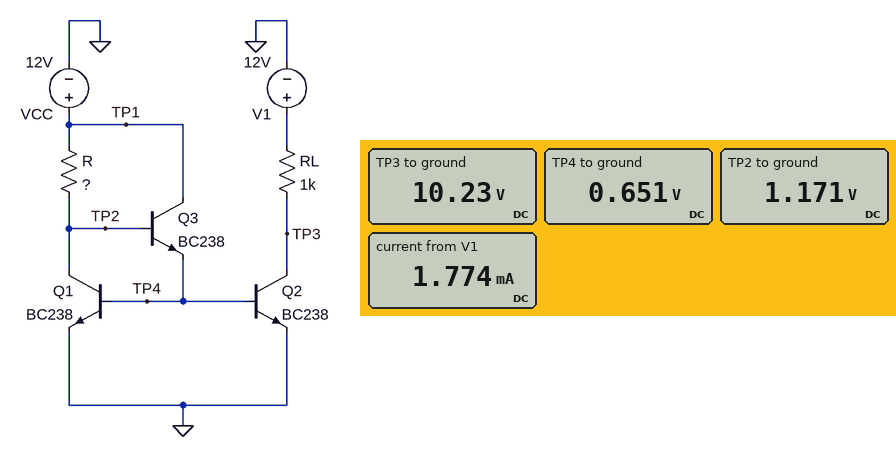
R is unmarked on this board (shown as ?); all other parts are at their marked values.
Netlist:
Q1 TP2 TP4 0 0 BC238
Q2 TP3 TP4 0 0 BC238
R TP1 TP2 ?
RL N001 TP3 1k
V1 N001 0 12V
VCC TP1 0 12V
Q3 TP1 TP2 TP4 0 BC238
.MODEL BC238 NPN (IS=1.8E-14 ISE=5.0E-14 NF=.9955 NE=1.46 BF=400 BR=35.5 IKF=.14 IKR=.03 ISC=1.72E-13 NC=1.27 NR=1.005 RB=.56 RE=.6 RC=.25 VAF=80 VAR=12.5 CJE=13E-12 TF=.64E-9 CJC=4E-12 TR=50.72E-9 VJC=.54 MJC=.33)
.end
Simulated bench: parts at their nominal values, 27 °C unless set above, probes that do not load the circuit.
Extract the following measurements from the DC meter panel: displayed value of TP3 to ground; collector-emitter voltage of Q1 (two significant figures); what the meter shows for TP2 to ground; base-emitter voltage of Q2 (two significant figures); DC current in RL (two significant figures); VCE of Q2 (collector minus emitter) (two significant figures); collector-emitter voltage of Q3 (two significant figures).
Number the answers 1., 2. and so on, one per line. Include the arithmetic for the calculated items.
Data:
1. 10.23 V
2. 1.171 V = 1.2 V
3. 1.171 V
4. 651 mV = 650 mV
5. (12 V - 10.23 V) / 1 kΩ = 1.8 mA
6. 10.23 V = 10 V
7. 12 V - 651 mV = 11 V
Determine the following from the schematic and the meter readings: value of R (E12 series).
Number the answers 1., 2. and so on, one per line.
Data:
1. 6.8 kΩ
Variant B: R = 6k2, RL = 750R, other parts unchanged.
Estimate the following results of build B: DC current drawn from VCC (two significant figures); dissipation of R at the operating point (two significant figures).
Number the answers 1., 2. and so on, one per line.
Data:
1. 1.8 mA
2. 19 mW
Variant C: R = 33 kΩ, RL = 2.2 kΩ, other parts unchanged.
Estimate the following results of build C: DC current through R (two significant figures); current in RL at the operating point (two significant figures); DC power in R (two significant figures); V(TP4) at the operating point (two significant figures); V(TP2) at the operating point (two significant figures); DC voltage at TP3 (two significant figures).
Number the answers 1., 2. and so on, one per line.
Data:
1. 330 µA
2. 370 µA
3. 3.6 mW
4. 610 mV
5. 1.1 V
6. 11 V
